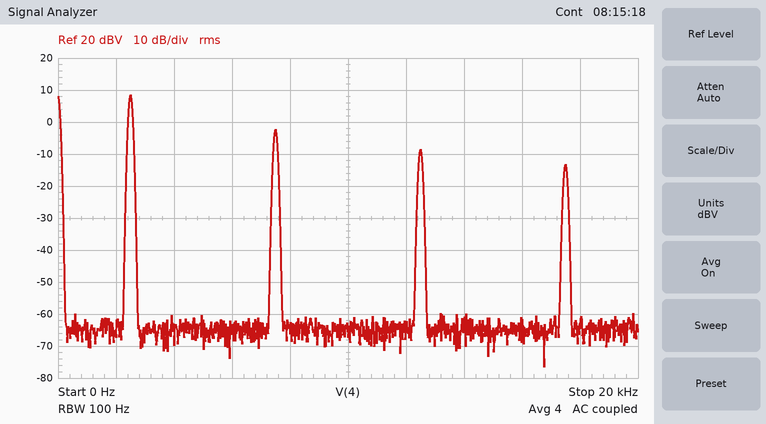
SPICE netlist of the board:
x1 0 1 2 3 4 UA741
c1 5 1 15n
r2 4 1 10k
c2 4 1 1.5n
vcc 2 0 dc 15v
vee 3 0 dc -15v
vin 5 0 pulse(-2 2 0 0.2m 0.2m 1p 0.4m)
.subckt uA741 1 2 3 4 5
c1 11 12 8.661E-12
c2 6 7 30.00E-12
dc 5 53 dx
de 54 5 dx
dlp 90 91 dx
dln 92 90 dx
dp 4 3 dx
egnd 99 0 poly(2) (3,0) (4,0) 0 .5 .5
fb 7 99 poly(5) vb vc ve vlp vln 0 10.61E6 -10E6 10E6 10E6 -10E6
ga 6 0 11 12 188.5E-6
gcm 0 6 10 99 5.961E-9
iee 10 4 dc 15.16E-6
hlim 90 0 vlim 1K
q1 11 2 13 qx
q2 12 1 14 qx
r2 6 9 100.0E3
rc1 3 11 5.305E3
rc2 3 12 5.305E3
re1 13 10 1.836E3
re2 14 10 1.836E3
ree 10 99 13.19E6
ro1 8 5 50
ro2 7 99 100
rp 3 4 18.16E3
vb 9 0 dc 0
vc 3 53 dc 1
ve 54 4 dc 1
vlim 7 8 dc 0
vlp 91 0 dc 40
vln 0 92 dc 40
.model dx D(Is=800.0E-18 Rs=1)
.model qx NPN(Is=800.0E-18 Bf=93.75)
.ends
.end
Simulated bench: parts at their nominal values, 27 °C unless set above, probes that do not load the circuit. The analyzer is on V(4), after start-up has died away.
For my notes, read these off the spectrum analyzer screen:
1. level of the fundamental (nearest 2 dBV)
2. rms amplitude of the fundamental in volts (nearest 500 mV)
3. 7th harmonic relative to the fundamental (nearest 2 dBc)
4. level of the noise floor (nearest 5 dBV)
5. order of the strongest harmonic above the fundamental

8 dBV
2.5 V
-22 dBc
-65 dBV
3
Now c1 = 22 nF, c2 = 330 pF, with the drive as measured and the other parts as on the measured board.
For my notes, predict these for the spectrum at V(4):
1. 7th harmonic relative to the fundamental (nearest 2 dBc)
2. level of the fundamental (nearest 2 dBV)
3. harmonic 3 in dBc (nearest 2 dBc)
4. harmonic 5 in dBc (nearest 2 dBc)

-12 dBc
12 dBV
-8 dBc
-10 dBc
